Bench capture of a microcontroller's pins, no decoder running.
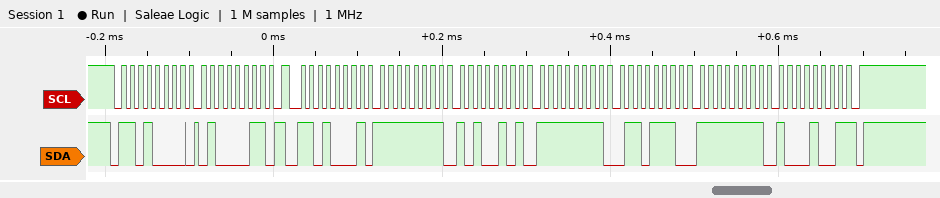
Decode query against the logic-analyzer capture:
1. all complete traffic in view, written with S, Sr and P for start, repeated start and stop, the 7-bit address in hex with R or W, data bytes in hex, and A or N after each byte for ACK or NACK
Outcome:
S 68W A 43 A Sr 68R A FF A A5 A FF A 6E A FF A 89 N P
